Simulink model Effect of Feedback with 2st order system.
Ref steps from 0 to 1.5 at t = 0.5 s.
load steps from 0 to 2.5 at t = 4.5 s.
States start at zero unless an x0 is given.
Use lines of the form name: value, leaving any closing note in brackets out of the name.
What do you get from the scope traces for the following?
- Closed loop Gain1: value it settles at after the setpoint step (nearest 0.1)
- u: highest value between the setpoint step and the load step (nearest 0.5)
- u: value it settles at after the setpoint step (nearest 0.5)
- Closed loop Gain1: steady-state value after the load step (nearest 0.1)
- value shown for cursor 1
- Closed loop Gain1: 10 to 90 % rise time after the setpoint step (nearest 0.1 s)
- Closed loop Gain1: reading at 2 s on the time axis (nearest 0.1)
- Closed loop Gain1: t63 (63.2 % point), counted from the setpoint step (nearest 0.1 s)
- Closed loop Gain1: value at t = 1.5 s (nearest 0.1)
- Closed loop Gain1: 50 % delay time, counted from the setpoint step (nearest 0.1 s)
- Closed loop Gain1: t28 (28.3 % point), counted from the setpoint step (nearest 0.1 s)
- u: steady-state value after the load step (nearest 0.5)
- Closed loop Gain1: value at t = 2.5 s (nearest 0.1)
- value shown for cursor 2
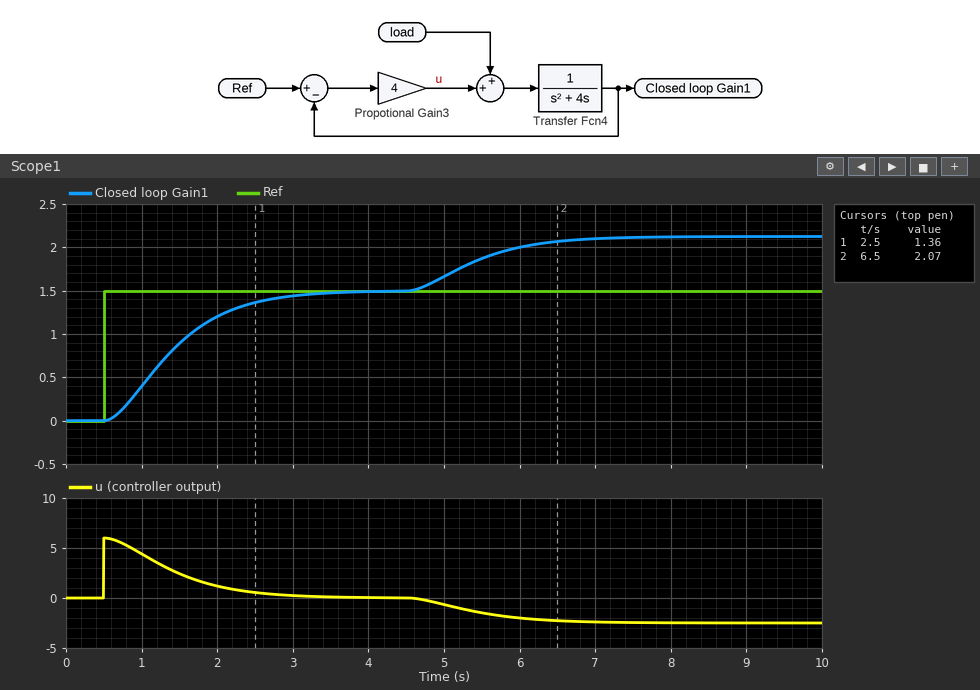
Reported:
Closed loop Gain1: value it settles at after the setpoint step: 1.5
u: highest value between the setpoint step and the load step: 6.0
u: value it settles at after the setpoint step: 0.0
Closed loop Gain1: steady-state value after the load step: 2.1
value shown for cursor 1: 1.36
Closed loop Gain1: 10 to 90 % rise time after the setpoint step: 1.7 s
Closed loop Gain1: reading at 2 s on the time axis: 1.2
Closed loop Gain1: t63 (63.2 % point), counted from the setpoint step: 1.1 s
Closed loop Gain1: value at t = 1.5 s: 0.9
Closed loop Gain1: 50 % delay time, counted from the setpoint step: 0.8 s
Closed loop Gain1: t28 (28.3 % point), counted from the setpoint step: 0.5 s
u: steady-state value after the load step: -2.5
Closed loop Gain1: value at t = 2.5 s: 1.4
value shown for cursor 2: 2.07
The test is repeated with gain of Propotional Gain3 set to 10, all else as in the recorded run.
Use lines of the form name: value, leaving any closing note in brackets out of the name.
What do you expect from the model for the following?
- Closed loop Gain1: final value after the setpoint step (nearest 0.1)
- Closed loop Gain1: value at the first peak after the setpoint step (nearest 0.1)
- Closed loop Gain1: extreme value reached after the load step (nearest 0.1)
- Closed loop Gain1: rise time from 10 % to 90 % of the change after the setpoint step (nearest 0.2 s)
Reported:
Closed loop Gain1: final value after the setpoint step: 1.5
Closed loop Gain1: value at the first peak after the setpoint step: 1.6
Closed loop Gain1: extreme value reached after the load step: 1.8
Closed loop Gain1: rise time from 10 % to 90 % of the change after the setpoint step: 0.6 s
